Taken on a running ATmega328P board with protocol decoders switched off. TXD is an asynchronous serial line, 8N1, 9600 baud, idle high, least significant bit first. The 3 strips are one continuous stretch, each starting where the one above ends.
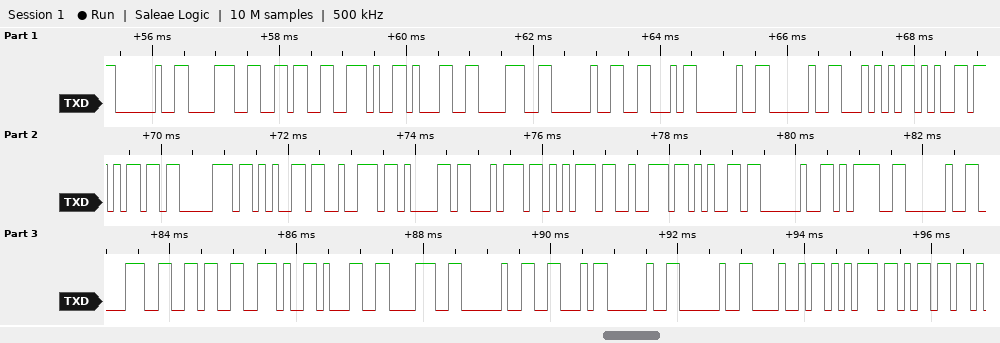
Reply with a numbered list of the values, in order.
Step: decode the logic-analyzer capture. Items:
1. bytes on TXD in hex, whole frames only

1. 20 38 36 2E 31 38 20 46 20 20 54 65 6D 70 65 72 61 74 75 72 65 20 3D 20 38 36 2E 31 38 20 46 20 20 48 75 6D
